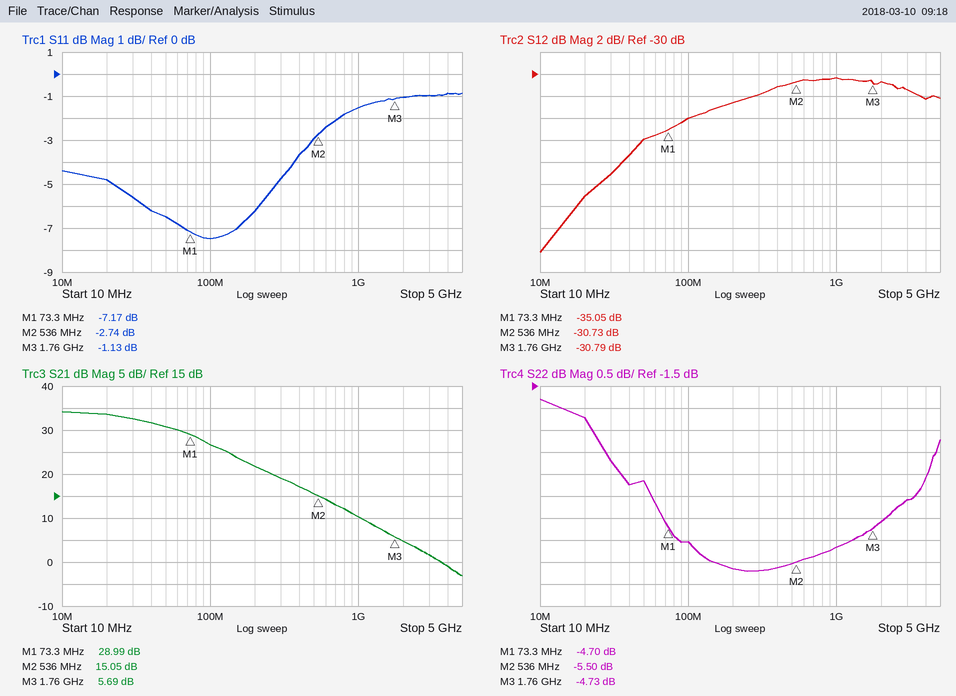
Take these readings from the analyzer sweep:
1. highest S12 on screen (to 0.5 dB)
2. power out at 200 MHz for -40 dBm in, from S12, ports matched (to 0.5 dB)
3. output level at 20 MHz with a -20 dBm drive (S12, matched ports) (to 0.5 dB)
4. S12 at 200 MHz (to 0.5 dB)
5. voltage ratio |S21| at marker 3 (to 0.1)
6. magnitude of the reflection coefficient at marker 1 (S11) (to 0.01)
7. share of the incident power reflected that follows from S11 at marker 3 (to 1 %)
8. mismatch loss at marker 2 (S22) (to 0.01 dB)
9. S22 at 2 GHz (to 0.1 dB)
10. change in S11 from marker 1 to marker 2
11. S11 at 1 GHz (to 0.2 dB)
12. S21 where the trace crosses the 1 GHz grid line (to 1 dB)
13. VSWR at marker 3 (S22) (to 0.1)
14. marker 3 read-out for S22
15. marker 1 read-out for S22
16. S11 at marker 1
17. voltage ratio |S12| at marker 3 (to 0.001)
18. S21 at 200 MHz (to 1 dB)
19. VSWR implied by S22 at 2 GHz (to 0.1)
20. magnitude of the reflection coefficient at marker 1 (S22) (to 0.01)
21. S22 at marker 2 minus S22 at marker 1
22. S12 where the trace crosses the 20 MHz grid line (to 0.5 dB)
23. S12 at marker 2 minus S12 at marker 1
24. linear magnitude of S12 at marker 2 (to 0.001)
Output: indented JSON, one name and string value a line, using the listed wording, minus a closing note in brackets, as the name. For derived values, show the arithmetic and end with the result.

{
  "highest S12 on screen": "-30.5 dB",
  "power out at 200 MHz for -40 dBm in, from S12, ports matched": "-40 dBm + (-32.5 dB) = -72.5 dBm",
  "output level at 20 MHz with a -20 dBm drive (S12, matched ports)": "-20 dBm + (-41.0 dB) = -61.0 dBm",
  "S12 at 200 MHz": "-32.5 dB",
  "voltage ratio |S21| at marker 3": "10^(5.69/20) ≈ 1.9",
  "magnitude of the reflection coefficient at marker 1 (S11)": "10^(-7.17/20) ≈ 0.44",
  "share of the incident power reflected that follows from S11 at marker 3": "10^(-1.13/10) ≈ 77 %",
  "mismatch loss at marker 2 (S22)": "−10 log10(1 − 10^(-5.5/10)) ≈ 1.44 dB",
  "S22 at 2 GHz": "-4.6 dB",
  "change in S11 from marker 1 to marker 2": "-2.74 − (-7.17) = 4.43 dB",
  "S11 at 1 GHz": "-1.6 dB",
  "S21 where the trace crosses the 1 GHz grid line": "10 dB",
  "VSWR at marker 3 (S22)": "(1 + 0.5801)/(1 − 0.5801) ≈ 3.8",
  "marker 3 read-out for S22": "-4.73 dB",
  "marker 1 read-out for S22": "-4.70 dB",
  "S11 at marker 1": "-7.17 dB",
  "voltage ratio |S12| at marker 3": "10^(-30.79/20) ≈ 0.029",
  "S21 at 200 MHz": "22 dB",
  "VSWR implied by S22 at 2 GHz": "|Γ| = 10^(-4.6/20) = 0.5888; VSWR = (1 + 0.5888)/(1 − 0.5888) ≈ 3.9",
  "magnitude of the reflection coefficient at marker 1 (S22)": "10^(-4.7/20) ≈ 0.58",
  "S22 at marker 2 minus S22 at marker 1": "-5.5 − (-4.7) = -0.80 dB",
  "S12 where the trace crosses the 20 MHz grid line": "-41.0 dB",
  "S12 at marker 2 minus S12 at marker 1": "-30.73 − (-35.05) = 4.32 dB",
  "linear magnitude of S12 at marker 2": "10^(-30.73/20) ≈ 0.029"
}
